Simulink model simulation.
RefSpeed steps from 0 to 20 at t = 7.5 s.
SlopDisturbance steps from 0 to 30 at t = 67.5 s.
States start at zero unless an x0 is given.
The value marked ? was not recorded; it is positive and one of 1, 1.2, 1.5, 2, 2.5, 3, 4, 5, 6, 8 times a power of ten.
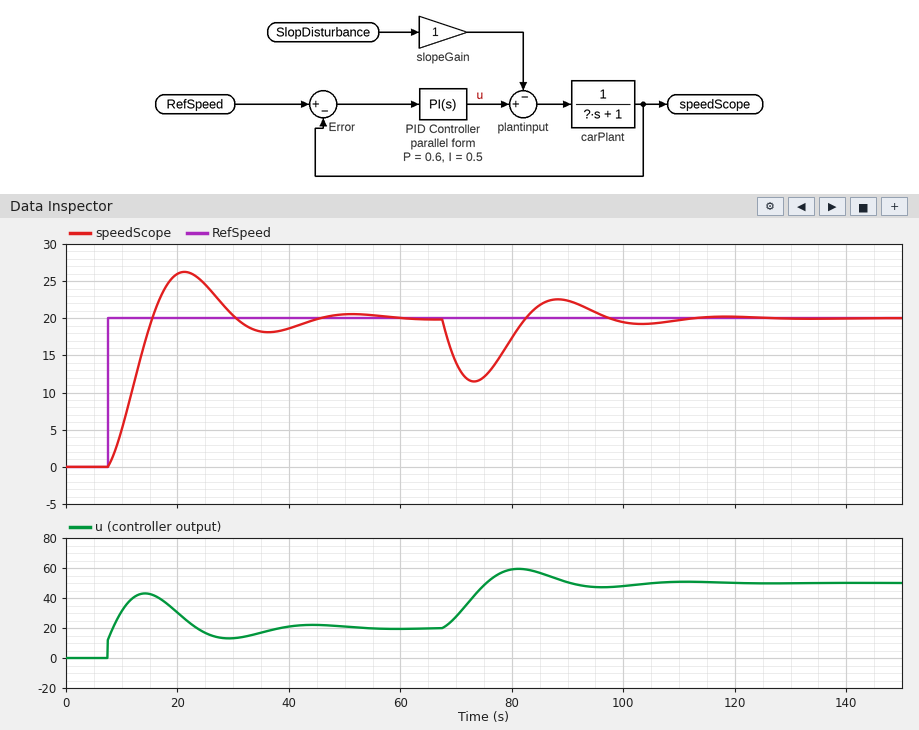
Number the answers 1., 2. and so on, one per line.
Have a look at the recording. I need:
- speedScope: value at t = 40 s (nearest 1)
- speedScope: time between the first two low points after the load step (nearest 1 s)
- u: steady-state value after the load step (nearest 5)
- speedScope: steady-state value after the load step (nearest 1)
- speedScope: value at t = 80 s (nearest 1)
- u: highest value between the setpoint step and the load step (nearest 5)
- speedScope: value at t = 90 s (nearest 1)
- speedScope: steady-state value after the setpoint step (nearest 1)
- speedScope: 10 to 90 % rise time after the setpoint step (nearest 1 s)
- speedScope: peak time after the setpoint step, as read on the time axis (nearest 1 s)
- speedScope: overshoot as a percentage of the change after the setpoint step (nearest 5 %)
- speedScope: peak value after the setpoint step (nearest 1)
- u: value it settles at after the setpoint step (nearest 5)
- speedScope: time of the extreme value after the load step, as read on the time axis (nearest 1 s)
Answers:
1. 19
2. 30 s
3. 50
4. 20
5. 17
6. 45
7. 22
8. 20
9. 6 s
10. 21 s
11. 30 %
12. 26
13. 20
14. 73 s
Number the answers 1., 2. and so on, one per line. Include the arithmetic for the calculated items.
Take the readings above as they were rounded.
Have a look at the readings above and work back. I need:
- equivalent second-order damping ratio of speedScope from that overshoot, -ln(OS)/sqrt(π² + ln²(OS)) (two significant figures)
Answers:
1. ln(0.3) = -1.204; 1.204 / sqrt(9.870 + 1.450) = 0.36
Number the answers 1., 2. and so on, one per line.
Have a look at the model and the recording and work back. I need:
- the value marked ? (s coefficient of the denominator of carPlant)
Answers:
1. 10
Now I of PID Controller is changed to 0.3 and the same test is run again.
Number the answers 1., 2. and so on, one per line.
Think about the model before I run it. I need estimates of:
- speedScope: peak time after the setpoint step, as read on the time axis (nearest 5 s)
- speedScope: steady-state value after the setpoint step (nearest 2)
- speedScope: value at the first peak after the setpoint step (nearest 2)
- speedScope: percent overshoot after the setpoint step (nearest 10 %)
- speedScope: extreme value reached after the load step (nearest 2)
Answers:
1. 25 s
2. 20
3. 24
4. 20 %
5. 10
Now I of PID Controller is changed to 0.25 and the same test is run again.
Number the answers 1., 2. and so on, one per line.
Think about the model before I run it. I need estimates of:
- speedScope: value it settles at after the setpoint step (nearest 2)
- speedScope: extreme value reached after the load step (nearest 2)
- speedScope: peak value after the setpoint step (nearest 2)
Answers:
1. 20
2. 10
3. 24
